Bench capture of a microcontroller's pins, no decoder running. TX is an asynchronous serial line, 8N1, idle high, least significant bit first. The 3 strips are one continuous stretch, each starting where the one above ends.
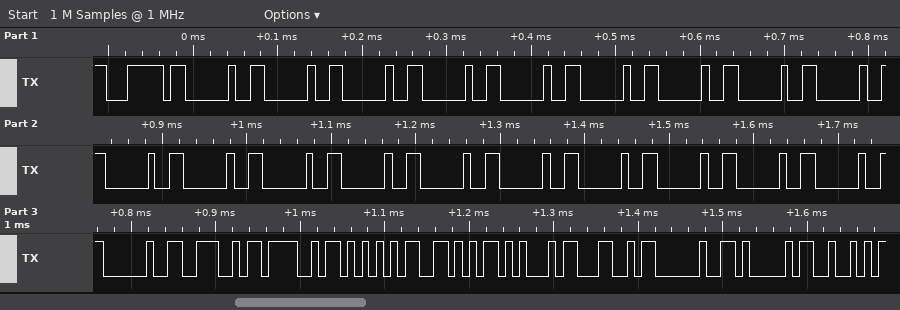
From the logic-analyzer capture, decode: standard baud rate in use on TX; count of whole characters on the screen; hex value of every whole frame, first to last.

115200 baud
30
7C 20 20 20 20 20 20 20 20 20 20 20 20 20 20 20 20 20 20 20 20 4E 4F 55 56 45 4C 20 41 52
